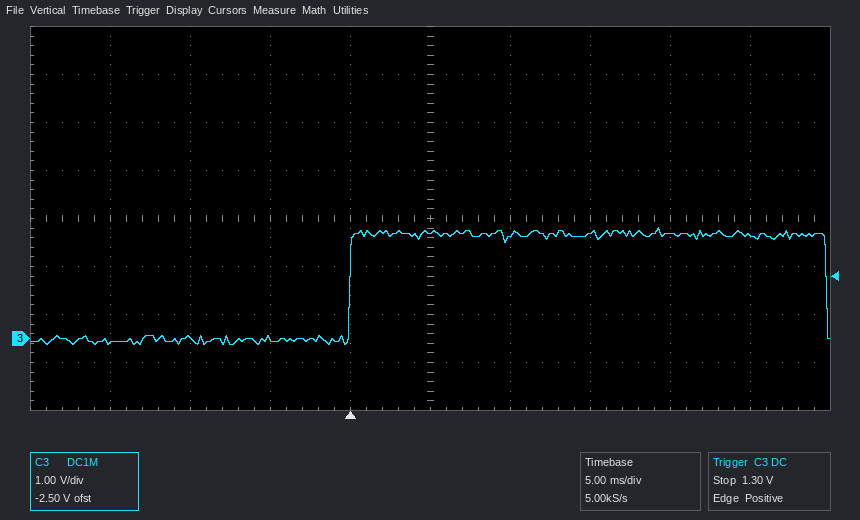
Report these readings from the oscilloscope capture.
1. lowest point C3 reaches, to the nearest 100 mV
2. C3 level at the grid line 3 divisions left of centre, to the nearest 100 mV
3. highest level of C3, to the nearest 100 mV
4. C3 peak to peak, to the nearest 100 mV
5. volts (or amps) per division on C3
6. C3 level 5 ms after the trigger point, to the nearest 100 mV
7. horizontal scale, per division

-100 mV
0.0 V
2.3 V
2.4 V
1 V
2.2 V
5 ms
